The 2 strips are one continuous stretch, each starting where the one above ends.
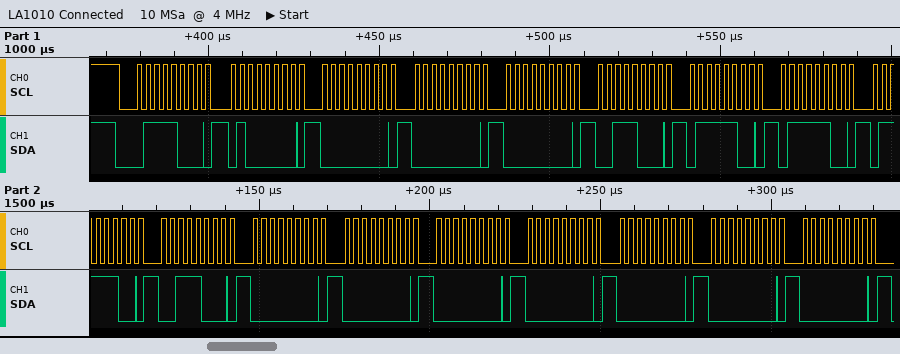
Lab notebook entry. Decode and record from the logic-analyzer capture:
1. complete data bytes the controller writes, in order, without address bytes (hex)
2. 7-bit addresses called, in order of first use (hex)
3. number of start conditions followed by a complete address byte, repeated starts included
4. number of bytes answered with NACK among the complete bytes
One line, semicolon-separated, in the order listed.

40 00 00 00 38 7C 7C 7C 38 00 00 00 00 00 00 00; 0x3C; 1; 0
